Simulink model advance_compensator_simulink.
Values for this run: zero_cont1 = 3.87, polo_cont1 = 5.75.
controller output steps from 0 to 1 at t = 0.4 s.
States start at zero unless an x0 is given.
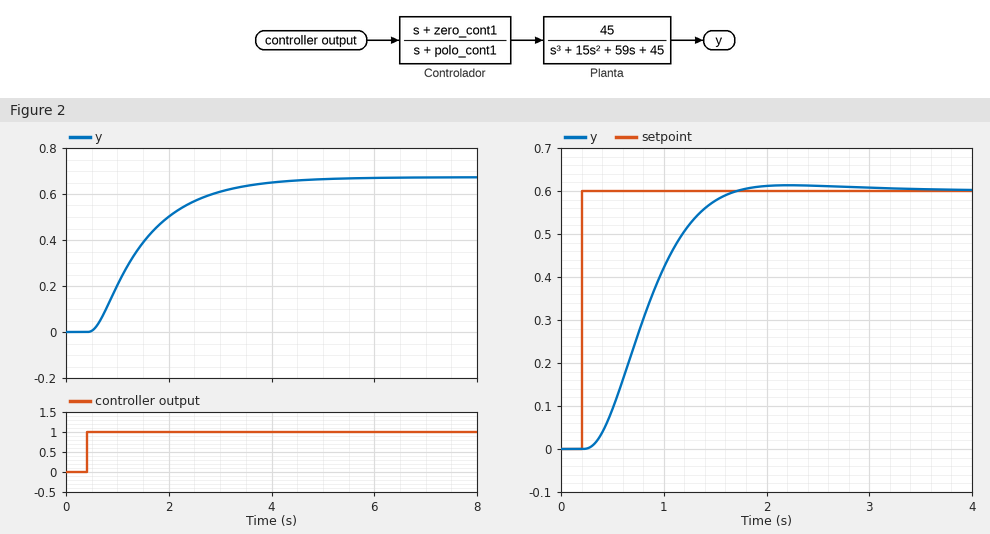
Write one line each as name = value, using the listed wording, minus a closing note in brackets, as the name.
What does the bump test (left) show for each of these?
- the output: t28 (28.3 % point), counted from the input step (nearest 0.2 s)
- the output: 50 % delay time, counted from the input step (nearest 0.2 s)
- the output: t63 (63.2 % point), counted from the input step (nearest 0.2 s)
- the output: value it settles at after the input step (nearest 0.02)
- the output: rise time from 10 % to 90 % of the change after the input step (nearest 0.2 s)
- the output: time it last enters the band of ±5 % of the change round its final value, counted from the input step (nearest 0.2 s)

the output: t28 (28.3 % point), counted from the input step = 0.6 s
the output: 50 % delay time, counted from the input step = 1.0 s
the output: t63 (63.2 % point), counted from the input step = 1.2 s
the output: value it settles at after the input step = 0.68
the output: rise time from 10 % to 90 % of the change after the input step = 2.2 s
the output: time it last enters the band of ±5 % of the change round its final value, counted from the input step = 3.2 s
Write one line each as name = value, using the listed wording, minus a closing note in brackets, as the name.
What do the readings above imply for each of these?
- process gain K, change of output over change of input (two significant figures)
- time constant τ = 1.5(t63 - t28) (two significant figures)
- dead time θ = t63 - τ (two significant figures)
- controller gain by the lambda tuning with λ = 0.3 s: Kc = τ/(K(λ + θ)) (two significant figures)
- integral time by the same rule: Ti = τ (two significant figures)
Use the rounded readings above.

process gain K, change of output over change of input = 0.68
time constant τ = 1.5(t63 - t28) = 0.90 s
dead time θ = t63 - τ = 0.30 s
controller gain by the lambda tuning with λ = 0.3 s: Kc = τ/(K(λ + θ)) = 2.2
integral time by the same rule: Ti = τ = 0.90 s
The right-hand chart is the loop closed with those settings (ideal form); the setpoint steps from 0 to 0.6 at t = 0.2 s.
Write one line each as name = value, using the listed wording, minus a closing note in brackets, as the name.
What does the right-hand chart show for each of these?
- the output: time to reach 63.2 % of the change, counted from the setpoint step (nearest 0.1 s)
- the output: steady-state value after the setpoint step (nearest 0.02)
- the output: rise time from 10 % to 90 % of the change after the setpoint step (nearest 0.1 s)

the output: time to reach 63.2 % of the change, counted from the setpoint step = 0.7 s
the output: steady-state value after the setpoint step = 0.60
the output: rise time from 10 % to 90 % of the change after the setpoint step = 0.9 s
